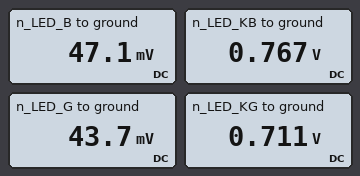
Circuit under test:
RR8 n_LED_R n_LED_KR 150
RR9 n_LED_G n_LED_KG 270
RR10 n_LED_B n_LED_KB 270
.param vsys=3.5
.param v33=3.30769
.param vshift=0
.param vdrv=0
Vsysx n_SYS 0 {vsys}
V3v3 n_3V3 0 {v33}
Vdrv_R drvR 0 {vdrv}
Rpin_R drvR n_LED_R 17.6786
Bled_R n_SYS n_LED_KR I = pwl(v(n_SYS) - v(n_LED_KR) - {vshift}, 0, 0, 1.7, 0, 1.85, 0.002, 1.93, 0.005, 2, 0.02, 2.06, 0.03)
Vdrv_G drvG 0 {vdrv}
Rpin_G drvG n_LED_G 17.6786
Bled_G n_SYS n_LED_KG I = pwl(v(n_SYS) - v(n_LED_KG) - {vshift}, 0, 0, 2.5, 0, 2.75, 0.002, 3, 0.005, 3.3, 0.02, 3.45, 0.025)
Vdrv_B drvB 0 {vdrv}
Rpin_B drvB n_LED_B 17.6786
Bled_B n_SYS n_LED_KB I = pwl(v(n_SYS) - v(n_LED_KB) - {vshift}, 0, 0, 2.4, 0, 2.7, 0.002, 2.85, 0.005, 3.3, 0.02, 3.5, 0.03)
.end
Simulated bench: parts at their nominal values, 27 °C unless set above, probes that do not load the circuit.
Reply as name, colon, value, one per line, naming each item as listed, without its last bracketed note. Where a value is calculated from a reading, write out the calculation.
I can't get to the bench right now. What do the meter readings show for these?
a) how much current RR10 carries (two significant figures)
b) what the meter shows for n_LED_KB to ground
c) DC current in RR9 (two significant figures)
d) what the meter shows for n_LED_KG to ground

how much current RR10 carries: (767 mV - 47.1 mV) / 270 Ω = 2.7 mA
what the meter shows for n_LED_KB to ground: 0.767 V
DC current in RR9: (711 mV - 43.7 mV) / 270 Ω = 2.5 mA
what the meter shows for n_LED_KG to ground: 0.711 V
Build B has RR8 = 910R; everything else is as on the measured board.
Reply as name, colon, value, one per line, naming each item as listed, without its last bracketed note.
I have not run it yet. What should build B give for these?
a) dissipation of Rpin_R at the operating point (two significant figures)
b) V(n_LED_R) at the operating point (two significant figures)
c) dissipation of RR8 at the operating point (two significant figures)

dissipation of Rpin_R at the operating point: 57 µW
V(n_LED_R) at the operating point: 32 mV
dissipation of RR8 at the operating point: 2.9 mW
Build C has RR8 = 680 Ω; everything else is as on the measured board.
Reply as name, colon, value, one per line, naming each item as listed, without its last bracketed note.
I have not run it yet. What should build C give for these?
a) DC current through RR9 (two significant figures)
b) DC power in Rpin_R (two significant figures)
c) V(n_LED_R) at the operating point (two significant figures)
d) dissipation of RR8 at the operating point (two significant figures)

DC current through RR9: 2.5 mA
DC power in Rpin_R: 98 µW
V(n_LED_R) at the operating point: 42 mV
dissipation of RR8 at the operating point: 3.8 mW
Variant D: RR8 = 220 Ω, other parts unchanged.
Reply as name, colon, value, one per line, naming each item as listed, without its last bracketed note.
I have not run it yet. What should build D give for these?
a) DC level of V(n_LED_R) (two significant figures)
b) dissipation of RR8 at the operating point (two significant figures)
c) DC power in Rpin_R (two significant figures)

DC level of V(n_LED_R): 120 mV
dissipation of RR8 at the operating point: 9.5 mW
DC power in Rpin_R: 760 µW
